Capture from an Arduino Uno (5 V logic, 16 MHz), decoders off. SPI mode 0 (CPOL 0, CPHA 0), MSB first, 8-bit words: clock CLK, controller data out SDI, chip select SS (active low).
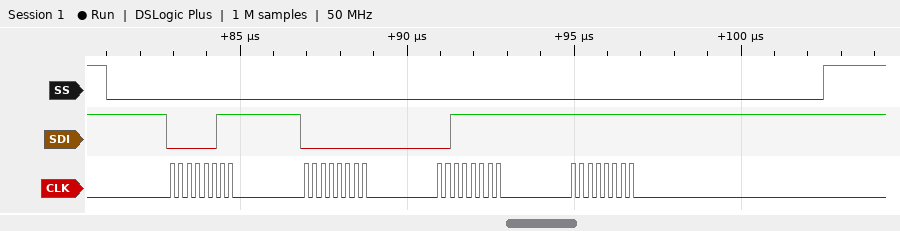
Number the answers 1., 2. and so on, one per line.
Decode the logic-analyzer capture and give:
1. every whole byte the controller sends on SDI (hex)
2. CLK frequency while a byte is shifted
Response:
1. 03 00 3F FF
2. 4 MHz
